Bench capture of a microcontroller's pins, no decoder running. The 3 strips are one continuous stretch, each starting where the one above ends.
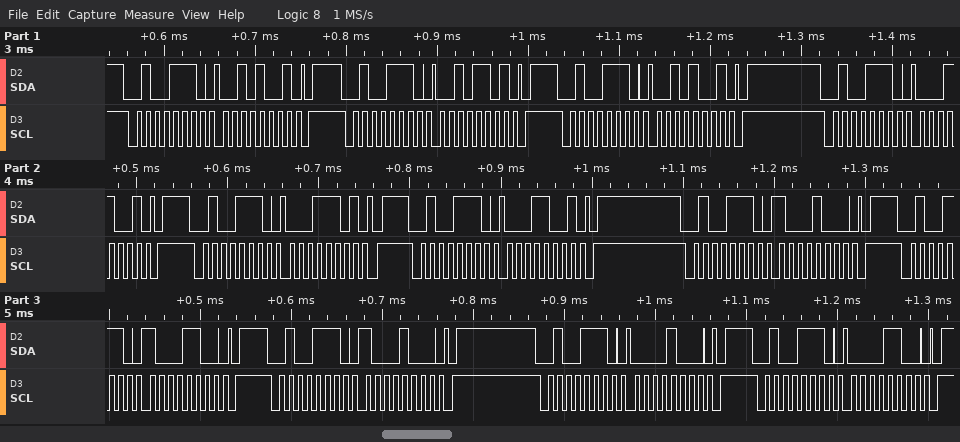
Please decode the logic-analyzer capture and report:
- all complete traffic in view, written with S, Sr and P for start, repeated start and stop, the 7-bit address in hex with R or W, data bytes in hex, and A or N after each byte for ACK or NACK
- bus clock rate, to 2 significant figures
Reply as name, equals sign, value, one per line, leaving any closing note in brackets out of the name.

all complete traffic in view, written with S, Sr and P for start, repeated start and stop, the 7-bit address in hex with R or W, data bytes in hex, and A or N after each byte for ACK or NACK = S 27W A 29 A P S 27W A 2D A P S 27W A 29 A P S 27W A 19 A P S 27W A 1D A P S 27W A 19 A P S 27W A 88 A P S 27W A 8C A P S 27W A 88 A P S 27W A 08 A P S 27W A 0C A P
bus clock rate, to 2 significant figures = 100 kHz
